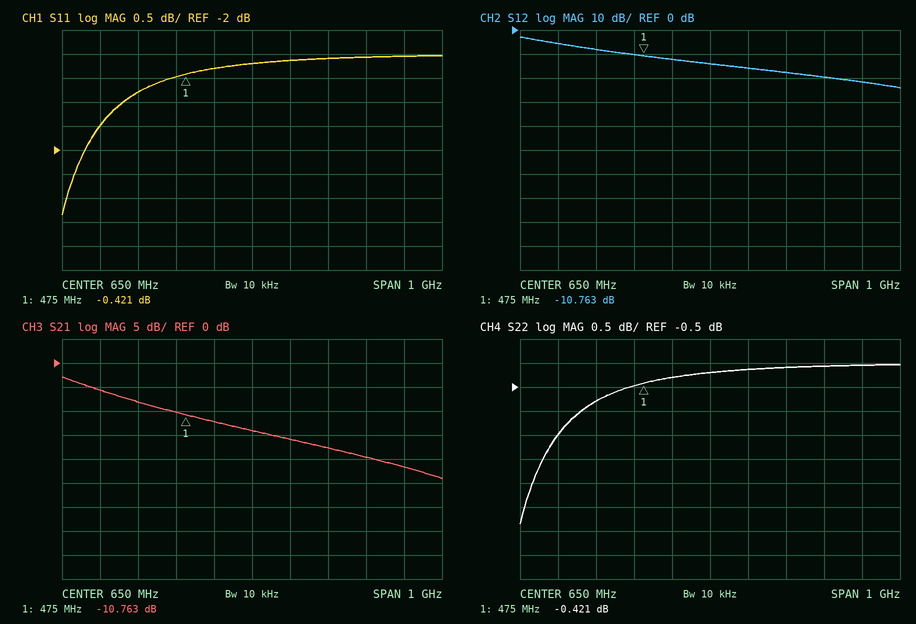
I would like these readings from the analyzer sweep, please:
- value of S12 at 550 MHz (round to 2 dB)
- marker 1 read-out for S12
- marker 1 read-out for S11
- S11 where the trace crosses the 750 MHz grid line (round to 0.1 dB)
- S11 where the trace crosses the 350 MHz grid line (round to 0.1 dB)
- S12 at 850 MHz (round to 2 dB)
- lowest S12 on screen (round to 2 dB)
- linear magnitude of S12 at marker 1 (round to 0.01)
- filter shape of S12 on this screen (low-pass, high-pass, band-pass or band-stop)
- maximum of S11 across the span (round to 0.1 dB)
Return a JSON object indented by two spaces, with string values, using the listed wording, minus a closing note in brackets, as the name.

{
  "value of S12 at 550 MHz": "-12 dB",
  "marker 1 read-out for S12": "-10.763 dB",
  "marker 1 read-out for S11": "-0.421 dB",
  "S11 where the trace crosses the 750 MHz grid line": "-0.1 dB",
  "S11 where the trace crosses the 350 MHz grid line": "-0.8 dB",
  "S12 at 850 MHz": "-18 dB",
  "lowest S12 on screen": "-24 dB",
  "linear magnitude of S12 at marker 1": "0.29",
  "filter shape of S12 on this screen": "low-pass",
  "maximum of S11 across the span": "0.0 dB"
}
